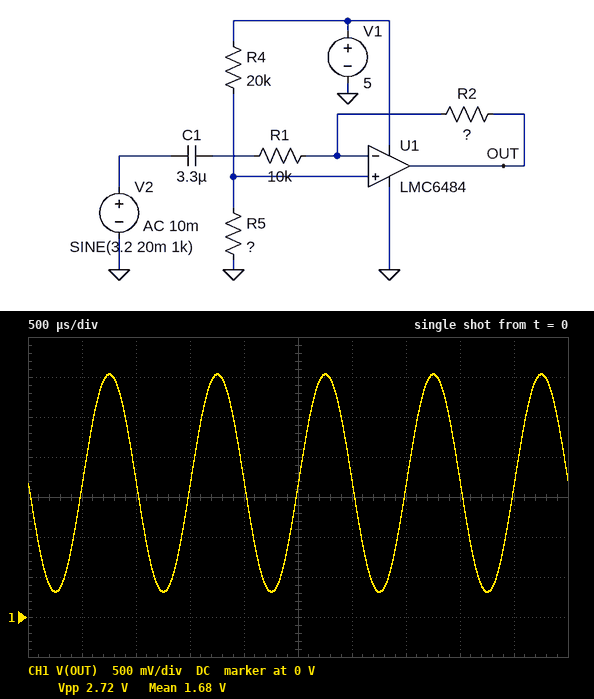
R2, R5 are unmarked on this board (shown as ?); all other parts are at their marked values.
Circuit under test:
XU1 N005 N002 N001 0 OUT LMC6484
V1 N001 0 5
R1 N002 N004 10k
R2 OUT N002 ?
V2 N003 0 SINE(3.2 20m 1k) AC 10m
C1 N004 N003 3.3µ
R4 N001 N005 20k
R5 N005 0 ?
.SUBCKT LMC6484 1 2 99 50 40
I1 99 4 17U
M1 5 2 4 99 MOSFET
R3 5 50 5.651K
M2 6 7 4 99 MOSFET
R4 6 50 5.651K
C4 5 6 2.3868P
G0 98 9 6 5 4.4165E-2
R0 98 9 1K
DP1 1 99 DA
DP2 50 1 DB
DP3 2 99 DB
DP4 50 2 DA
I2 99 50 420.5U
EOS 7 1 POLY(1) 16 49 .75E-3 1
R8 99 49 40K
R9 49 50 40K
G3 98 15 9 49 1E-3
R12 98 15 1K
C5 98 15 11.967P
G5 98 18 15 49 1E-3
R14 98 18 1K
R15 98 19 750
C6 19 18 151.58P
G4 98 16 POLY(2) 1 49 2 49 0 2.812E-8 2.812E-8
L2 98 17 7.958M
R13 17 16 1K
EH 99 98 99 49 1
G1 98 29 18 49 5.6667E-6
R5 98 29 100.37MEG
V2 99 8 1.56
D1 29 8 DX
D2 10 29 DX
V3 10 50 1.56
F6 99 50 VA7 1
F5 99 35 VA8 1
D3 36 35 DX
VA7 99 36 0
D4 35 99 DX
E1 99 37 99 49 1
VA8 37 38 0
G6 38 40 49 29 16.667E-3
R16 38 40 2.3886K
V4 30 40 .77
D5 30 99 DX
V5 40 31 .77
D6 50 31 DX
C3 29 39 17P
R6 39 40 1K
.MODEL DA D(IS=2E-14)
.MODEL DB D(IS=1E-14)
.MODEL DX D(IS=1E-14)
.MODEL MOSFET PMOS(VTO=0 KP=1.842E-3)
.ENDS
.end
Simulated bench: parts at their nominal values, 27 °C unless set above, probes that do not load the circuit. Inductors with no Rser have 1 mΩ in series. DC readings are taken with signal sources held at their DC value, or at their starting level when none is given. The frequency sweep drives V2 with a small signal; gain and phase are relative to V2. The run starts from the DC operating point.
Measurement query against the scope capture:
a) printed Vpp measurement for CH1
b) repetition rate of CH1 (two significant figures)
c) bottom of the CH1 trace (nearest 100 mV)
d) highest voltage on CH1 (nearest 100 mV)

2.72 V
1.0 kHz
300 mV
3.0 V
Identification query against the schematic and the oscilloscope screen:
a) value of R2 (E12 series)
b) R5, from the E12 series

680 kΩ
10 kΩ
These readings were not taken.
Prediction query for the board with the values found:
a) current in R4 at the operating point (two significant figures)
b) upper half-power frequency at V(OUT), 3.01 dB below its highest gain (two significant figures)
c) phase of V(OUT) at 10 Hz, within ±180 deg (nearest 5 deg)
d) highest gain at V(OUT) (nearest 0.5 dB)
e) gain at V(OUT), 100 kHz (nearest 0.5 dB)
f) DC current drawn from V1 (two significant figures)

170 µA
34 kHz
-155 deg
36.5 dB
27.0 dB
670 µA
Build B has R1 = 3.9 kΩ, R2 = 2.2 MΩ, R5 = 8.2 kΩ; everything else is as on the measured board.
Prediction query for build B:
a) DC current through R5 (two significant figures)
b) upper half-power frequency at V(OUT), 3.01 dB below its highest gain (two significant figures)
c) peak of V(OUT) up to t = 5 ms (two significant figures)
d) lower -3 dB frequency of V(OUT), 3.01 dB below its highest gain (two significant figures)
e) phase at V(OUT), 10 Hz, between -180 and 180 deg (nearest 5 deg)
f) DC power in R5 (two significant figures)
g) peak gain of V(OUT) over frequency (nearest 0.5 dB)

180 µA
4.1 kHz
5.0 V
12 Hz
-130 deg
260 µW
55.0 dB
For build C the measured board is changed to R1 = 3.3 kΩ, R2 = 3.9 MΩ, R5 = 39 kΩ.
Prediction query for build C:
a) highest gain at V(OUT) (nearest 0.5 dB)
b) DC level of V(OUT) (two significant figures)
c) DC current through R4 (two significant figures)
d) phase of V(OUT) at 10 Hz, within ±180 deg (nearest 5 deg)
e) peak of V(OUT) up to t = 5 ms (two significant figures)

61.5 dB
3.3 V
85 µA
-125 deg
5.0 V
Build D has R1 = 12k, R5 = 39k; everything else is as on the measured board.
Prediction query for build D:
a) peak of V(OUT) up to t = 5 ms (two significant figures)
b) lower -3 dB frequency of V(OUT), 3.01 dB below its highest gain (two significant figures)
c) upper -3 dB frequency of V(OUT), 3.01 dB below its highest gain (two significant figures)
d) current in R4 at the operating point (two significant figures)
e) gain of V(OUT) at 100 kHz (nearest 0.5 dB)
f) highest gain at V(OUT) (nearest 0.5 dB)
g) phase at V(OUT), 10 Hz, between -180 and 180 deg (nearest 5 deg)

4.4 V
4.0 Hz
41 kHz
85 µA
26.5 dB
35.0 dB
-160 deg
